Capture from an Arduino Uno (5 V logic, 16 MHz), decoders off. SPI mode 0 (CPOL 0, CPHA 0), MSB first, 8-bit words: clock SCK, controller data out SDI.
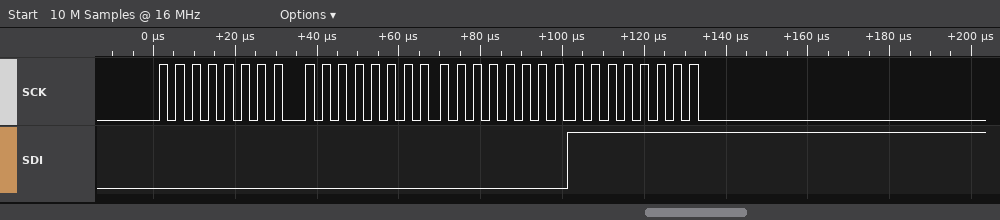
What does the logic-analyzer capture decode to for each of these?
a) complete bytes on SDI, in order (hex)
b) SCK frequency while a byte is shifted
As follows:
00 00 00 FF
250 kHz
